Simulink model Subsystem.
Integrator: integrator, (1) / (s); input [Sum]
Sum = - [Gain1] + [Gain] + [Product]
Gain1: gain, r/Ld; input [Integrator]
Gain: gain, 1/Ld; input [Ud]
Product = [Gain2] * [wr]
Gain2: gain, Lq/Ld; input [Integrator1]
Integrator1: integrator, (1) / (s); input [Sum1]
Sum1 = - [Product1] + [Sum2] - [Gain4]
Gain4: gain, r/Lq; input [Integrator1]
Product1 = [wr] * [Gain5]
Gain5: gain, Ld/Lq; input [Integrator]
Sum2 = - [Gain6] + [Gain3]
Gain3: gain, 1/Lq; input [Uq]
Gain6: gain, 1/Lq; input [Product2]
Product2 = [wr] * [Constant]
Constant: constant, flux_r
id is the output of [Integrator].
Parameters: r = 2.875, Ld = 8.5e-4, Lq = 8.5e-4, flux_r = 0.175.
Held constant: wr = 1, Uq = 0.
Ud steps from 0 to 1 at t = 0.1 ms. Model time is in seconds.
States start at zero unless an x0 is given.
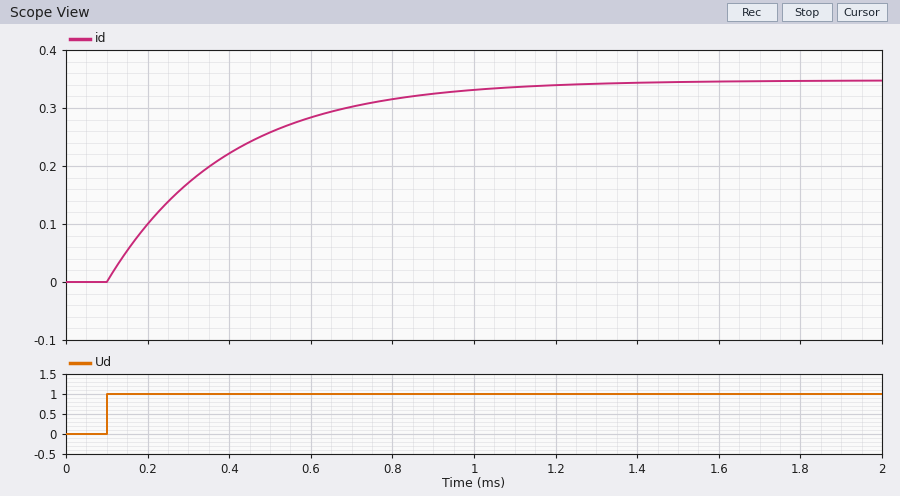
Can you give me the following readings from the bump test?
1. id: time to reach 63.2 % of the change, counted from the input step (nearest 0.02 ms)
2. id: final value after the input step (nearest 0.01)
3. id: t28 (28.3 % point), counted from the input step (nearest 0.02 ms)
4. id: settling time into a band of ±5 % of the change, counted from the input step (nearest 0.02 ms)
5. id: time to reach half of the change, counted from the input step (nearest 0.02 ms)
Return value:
0.30 ms
0.35
0.10 ms
0.88 ms
0.20 ms
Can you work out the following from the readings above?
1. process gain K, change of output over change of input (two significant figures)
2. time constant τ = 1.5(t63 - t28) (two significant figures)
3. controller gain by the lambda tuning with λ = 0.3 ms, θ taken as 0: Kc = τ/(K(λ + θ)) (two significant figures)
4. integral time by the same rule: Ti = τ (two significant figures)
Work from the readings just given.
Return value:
0.35
0.30 ms
2.9
0.30 ms
